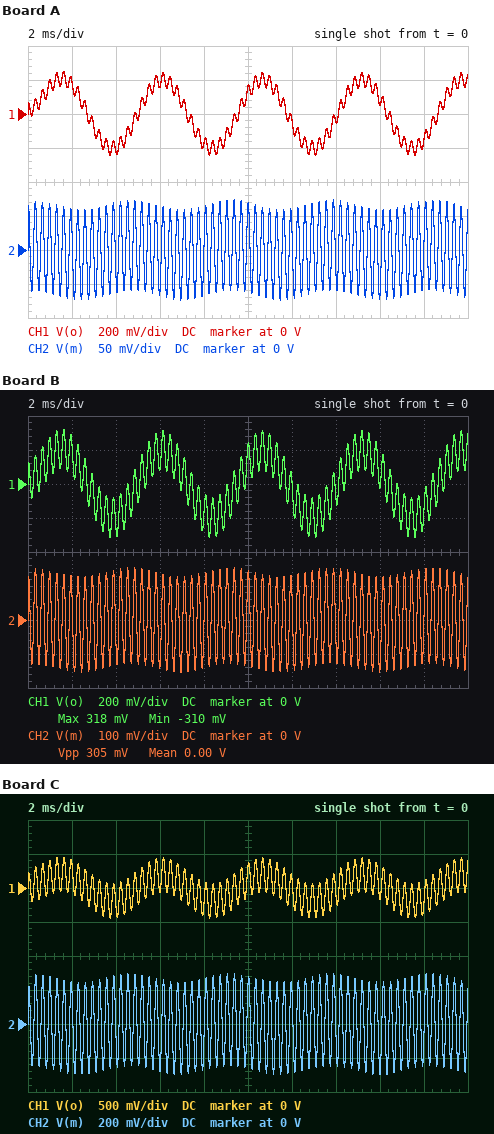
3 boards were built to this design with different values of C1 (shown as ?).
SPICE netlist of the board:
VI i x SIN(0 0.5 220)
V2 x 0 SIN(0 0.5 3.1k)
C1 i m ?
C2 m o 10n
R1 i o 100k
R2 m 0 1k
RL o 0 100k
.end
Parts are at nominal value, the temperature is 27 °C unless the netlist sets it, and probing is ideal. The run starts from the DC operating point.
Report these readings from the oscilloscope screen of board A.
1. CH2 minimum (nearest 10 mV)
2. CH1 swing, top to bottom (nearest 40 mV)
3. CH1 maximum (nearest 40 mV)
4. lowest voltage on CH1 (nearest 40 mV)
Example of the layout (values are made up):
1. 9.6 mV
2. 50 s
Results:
1. -70 mV
2. 480 mV
3. 240 mV
4. -240 mV
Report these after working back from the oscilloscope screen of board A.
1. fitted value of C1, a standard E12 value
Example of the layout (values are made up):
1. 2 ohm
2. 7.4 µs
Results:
1. 6.8 nF
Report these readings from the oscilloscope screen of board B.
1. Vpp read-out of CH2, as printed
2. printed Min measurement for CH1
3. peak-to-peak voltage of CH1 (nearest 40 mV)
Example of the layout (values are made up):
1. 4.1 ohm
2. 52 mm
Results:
1. 305 mV
2. -310 mV
3. 640 mV
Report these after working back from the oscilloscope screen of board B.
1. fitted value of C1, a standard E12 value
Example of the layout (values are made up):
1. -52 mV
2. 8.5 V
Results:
1. 15 nF
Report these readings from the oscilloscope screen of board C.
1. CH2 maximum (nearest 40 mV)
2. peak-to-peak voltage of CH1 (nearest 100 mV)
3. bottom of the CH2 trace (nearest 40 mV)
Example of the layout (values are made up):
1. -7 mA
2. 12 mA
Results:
1. 280 mV
2. 900 mV
3. -280 mV
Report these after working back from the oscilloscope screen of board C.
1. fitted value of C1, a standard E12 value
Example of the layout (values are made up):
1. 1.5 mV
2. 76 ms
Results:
1. 33 nF
